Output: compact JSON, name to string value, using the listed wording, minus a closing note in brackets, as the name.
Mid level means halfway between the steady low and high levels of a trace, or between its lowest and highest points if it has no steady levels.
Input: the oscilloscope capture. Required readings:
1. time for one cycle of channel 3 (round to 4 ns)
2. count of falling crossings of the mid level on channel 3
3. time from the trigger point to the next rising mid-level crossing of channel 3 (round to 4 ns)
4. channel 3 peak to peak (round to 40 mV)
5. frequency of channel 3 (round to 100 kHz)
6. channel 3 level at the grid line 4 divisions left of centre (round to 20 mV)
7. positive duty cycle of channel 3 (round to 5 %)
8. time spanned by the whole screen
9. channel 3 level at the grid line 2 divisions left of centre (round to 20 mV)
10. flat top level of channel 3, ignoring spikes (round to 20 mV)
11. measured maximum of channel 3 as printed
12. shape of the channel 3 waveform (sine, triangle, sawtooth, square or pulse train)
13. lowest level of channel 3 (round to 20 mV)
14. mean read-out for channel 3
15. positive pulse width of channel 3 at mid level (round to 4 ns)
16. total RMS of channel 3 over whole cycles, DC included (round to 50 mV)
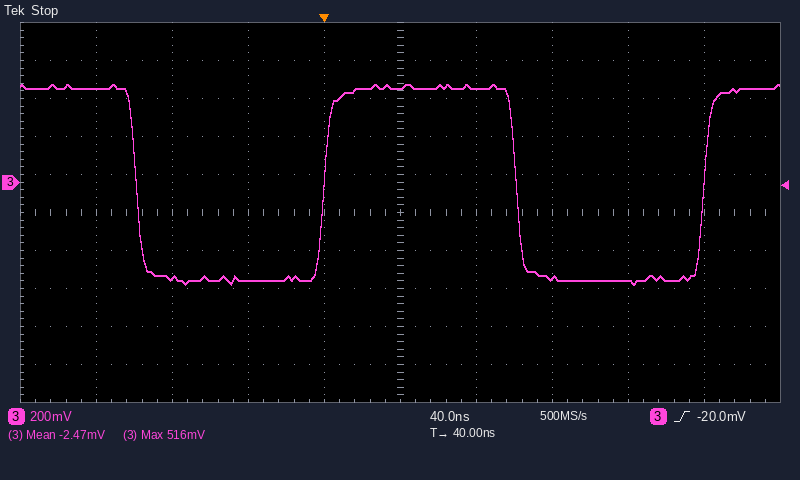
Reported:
{"time for one cycle of channel 3": "200 ns", "count of falling crossings of the mid level on channel 3": "2", "time from the trigger point to the next rising mid-level crossing of channel 3": "200 ns", "channel 3 peak to peak": "1.04 V", "frequency of channel 3": "5.0 MHz", "channel 3 level at the grid line 4 divisions left of centre": "500 mV", "positive duty cycle of channel 3": "50 %", "time spanned by the whole screen": "400 ns", "channel 3 level at the grid line 2 divisions left of centre": "-520 mV", "flat top level of channel 3, ignoring spikes": "500 mV", "measured maximum of channel 3 as printed": "516 mV", "shape of the channel 3 waveform": "square", "lowest level of channel 3": "-540 mV", "mean read-out for channel 3": "-2.47 mV", "positive pulse width of channel 3 at mid level": "100 ns", "total RMS of channel 3 over whole cycles, DC included": "500 mV"}
